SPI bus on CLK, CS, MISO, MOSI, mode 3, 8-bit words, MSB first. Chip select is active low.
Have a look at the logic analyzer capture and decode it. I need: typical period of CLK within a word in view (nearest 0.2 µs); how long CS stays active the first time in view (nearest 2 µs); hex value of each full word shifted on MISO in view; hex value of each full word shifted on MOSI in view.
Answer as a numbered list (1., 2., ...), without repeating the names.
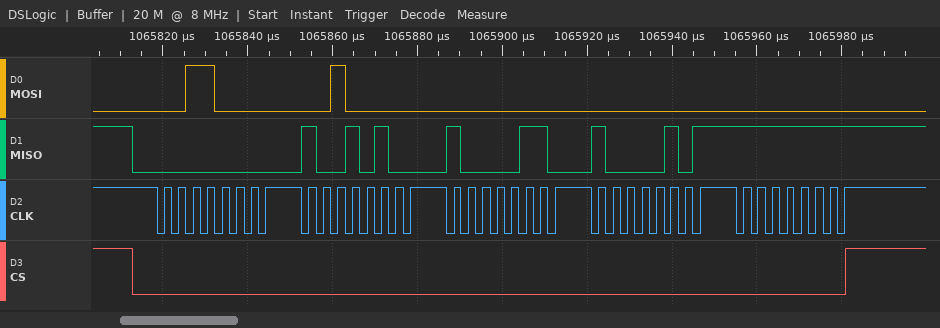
1. 3.4 µs
2. 168 µs
3. 00, 94, 86, 85, FF
4. 30, 20, 00, 00, 00
